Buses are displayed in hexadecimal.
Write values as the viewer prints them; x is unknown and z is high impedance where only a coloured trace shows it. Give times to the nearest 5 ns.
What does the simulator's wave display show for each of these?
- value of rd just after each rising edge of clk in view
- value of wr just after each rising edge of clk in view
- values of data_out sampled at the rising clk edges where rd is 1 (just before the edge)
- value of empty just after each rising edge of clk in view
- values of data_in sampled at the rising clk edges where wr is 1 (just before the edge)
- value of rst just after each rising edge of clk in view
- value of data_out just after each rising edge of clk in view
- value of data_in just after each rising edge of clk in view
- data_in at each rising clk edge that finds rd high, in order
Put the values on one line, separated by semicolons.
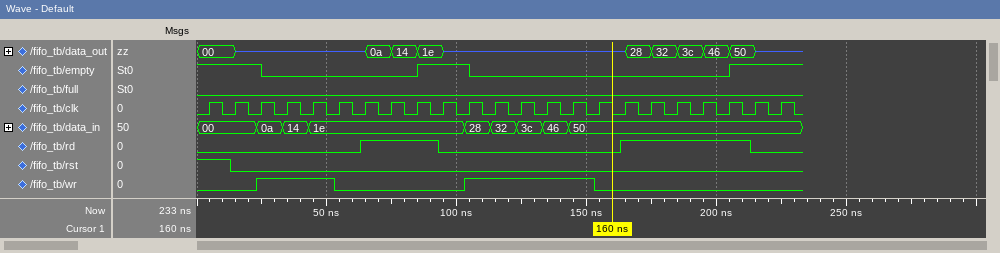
0 0 0 0 0 0 1 1 1 0 0 0 0 0 0 0 1 1 1 1 1 0 0; 0 0 1 1 1 0 0 0 0 0 1 1 1 1 1 0 0 0 0 0 0 0 0; z, 0a, 14, z, 28, 32, 3c, 46; 1 1 0 0 0 0 0 0 1 1 0 0 0 0 0 0 0 0 0 0 1 1 1; 0a, 14, 1e, 28, 32, 3c, 46, 50; 1 0 0 0 0 0 0 0 0 0 0 0 0 0 0 0 0 0 0 0 0 0 0; 00, z, z, z, z, z, 0a, 14, 1e, z, z, z, z, z, z, z, 28, 32, 3c, 46, 50, z, z; 00, 00, 0a, 14, 1e, 1e, 1e, 1e, 1e, 1e, 28, 32, 3c, 46, 50, 50, 50, 50, 50, 50, 50, 50, 50; 1e, 1e, 1e, 50, 50, 50, 50, 50
